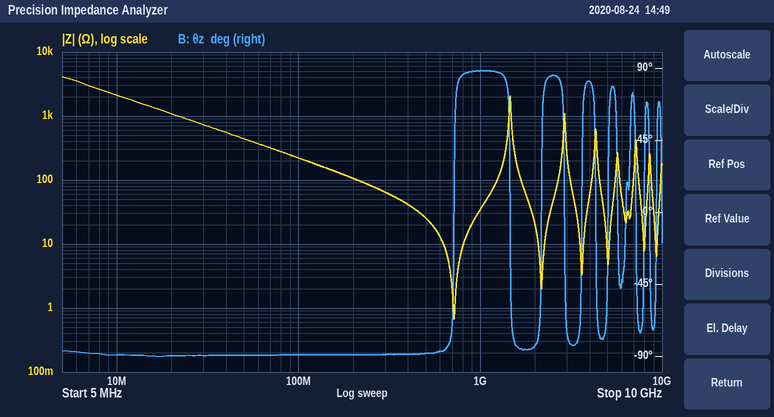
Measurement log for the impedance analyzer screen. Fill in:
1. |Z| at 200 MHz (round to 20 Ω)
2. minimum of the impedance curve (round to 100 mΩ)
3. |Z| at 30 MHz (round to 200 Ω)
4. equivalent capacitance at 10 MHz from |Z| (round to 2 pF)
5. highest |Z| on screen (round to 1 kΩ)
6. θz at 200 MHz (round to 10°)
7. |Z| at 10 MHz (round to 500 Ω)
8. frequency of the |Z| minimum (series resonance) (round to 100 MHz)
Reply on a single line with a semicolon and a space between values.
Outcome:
100 Ω; 700 mΩ; 800 Ω; 8 pF; 4 kΩ; -90°; 2.0 kΩ; 700 MHz
